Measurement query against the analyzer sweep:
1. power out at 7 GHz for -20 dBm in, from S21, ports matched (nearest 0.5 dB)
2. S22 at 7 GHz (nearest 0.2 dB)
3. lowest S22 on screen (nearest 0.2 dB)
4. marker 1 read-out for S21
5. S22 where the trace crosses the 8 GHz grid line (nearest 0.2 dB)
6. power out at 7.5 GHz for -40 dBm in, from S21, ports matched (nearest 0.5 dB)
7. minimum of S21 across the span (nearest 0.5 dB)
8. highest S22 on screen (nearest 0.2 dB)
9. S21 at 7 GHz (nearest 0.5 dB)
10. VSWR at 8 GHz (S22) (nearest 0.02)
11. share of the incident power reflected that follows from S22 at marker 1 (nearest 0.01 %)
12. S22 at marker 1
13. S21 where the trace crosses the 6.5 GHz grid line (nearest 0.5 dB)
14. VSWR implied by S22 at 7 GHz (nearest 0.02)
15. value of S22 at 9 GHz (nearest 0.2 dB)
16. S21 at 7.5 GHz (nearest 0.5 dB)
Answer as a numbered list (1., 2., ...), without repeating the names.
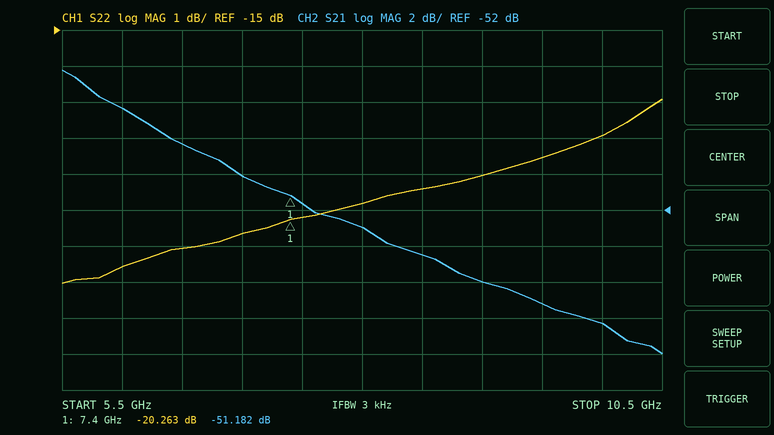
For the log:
1. -70.0 dBm
2. -20.6 dB
3. -22.0 dB
4. -51.182 dB
5. -19.8 dB
6. -91.5 dBm
7. -60.0 dB
8. -17.0 dB
9. -50.0 dB
10. 1.22
11. 0.94 %
12. -20.263 dB
13. -48.5 dB
14. 1.20
15. -19.0 dB
16. -51.5 dB
